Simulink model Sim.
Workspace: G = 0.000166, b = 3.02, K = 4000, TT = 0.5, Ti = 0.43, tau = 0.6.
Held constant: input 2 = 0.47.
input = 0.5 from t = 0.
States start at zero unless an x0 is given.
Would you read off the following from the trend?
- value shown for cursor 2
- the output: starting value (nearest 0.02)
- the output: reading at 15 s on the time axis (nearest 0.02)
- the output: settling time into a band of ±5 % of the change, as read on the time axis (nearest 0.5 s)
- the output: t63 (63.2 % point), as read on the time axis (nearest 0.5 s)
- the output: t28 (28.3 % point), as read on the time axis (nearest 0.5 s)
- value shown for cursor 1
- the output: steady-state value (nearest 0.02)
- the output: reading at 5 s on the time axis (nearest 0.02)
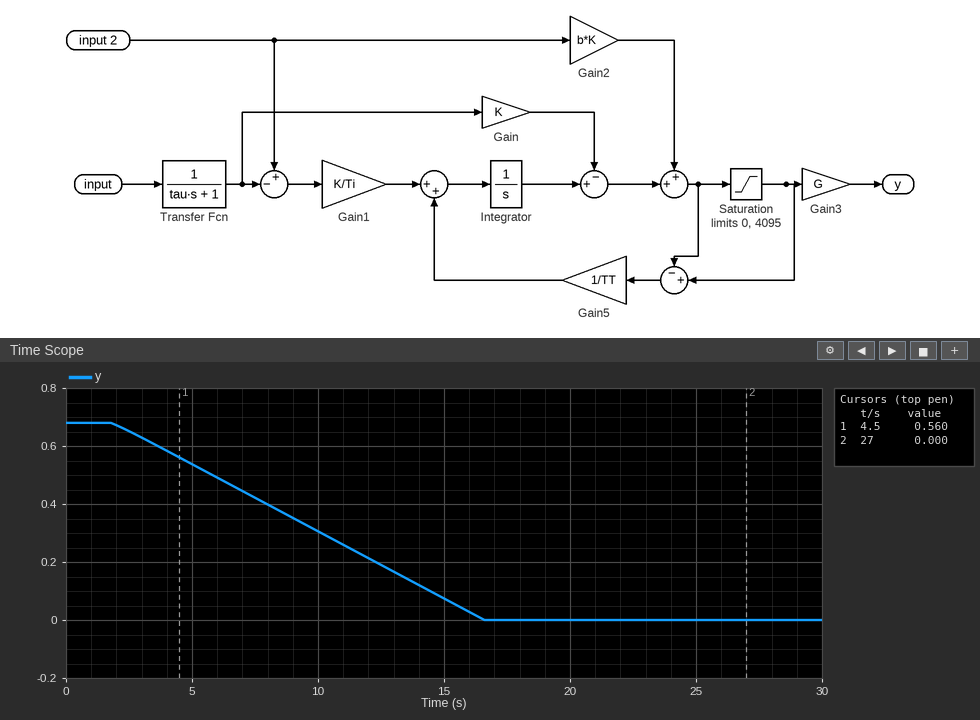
0.000
0.68
0.08
16.0 s
11.0 s
6.0 s
0.560
0.00
0.54
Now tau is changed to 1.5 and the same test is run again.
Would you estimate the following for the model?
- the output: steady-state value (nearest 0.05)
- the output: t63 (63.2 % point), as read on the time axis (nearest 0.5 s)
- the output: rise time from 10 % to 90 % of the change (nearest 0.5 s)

0.00
14.5 s
12.0 s
